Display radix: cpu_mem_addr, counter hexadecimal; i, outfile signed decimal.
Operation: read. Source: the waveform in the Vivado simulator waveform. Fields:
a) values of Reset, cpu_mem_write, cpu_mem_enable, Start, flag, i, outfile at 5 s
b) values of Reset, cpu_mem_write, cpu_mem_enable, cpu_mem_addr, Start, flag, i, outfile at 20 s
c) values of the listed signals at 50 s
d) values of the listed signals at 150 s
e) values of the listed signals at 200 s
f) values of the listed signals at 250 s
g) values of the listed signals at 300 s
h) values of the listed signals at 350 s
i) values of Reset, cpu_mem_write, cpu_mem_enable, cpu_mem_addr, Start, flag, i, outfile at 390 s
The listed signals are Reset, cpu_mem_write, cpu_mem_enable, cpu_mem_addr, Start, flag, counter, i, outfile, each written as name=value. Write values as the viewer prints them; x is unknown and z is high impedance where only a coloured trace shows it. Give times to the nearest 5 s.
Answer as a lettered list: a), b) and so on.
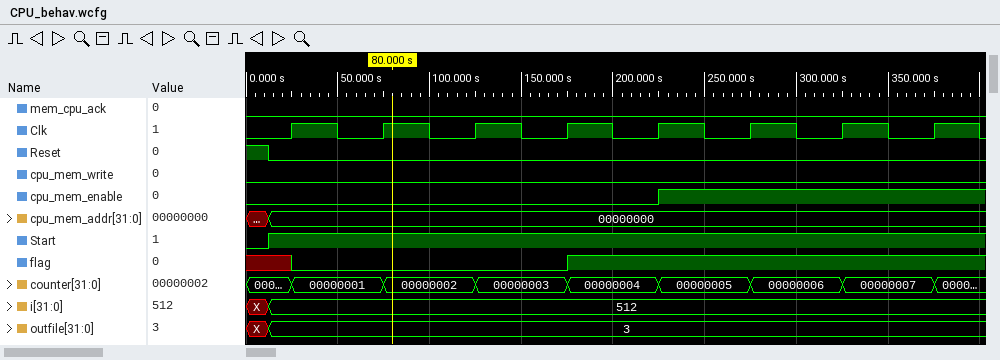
a) Reset=1, cpu_mem_write=0, cpu_mem_enable=0, Start=0, flag=x, i=X, outfile=X
b) Reset=0, cpu_mem_write=0, cpu_mem_enable=0, cpu_mem_addr=00000000, Start=1, flag=x, i=512, outfile=3
c) Reset=0, cpu_mem_write=0, cpu_mem_enable=0, cpu_mem_addr=00000000, Start=1, flag=0, counter=00000001, i=512, outfile=3
d) Reset=0, cpu_mem_write=0, cpu_mem_enable=0, cpu_mem_addr=00000000, Start=1, flag=0, counter=00000003, i=512, outfile=3
e) Reset=0, cpu_mem_write=0, cpu_mem_enable=0, cpu_mem_addr=00000000, Start=1, flag=1, counter=00000004, i=512, outfile=3
f) Reset=0, cpu_mem_write=0, cpu_mem_enable=1, cpu_mem_addr=00000000, Start=1, flag=1, counter=00000005, i=512, outfile=3
g) Reset=0, cpu_mem_write=0, cpu_mem_enable=1, cpu_mem_addr=00000000, Start=1, flag=1, counter=00000006, i=512, outfile=3
h) Reset=0, cpu_mem_write=0, cpu_mem_enable=1, cpu_mem_addr=00000000, Start=1, flag=1, counter=00000007, i=512, outfile=3
i) Reset=0, cpu_mem_write=0, cpu_mem_enable=1, cpu_mem_addr=00000000, Start=1, flag=1, i=512, outfile=3
